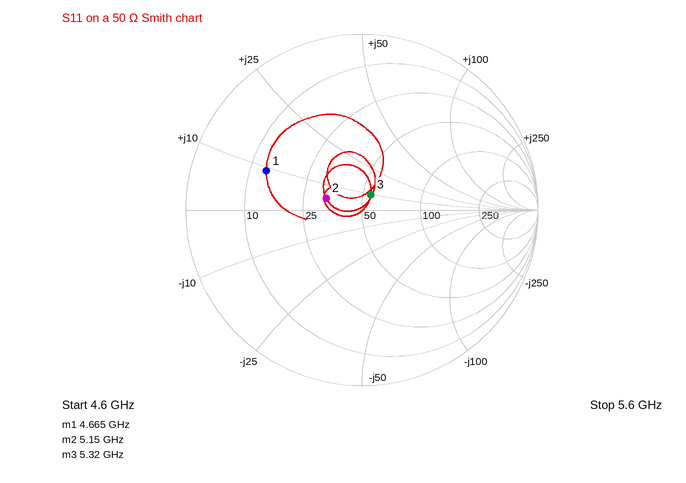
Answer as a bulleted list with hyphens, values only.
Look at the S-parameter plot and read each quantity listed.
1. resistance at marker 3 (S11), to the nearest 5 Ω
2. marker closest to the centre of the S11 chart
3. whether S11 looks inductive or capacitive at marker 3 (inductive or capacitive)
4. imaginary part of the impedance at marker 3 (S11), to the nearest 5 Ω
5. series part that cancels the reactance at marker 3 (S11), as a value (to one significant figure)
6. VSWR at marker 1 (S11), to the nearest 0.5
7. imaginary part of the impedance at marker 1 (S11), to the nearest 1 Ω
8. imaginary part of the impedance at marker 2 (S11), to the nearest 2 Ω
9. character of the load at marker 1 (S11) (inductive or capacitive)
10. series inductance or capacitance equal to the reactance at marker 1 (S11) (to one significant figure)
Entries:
- 55 Ω
- marker 3
- inductive
- +10 Ω
- 3 pF
- 4.0
- +9 Ω
- +4 Ω
- inductive
- 300 pH
